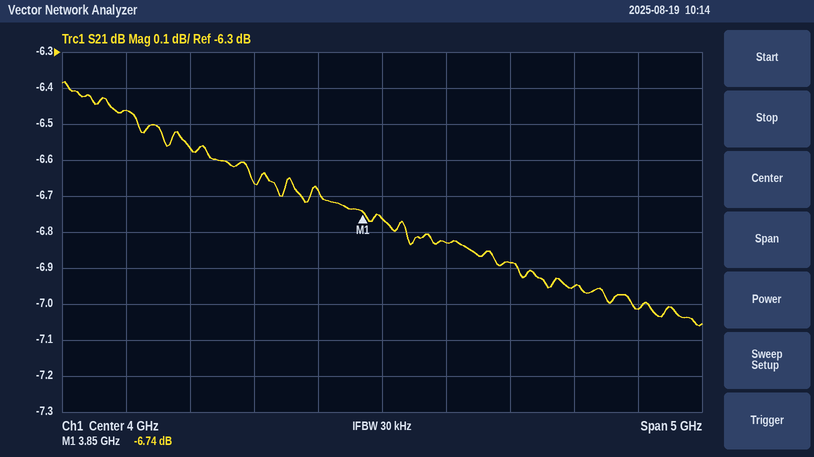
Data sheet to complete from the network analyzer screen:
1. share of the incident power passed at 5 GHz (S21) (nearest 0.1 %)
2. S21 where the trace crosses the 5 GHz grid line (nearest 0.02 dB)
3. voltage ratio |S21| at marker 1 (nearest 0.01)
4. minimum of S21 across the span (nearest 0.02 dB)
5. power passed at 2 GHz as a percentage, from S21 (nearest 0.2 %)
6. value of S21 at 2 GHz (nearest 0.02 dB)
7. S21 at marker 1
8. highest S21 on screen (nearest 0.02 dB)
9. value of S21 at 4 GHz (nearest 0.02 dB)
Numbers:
20.5 %
-6.88 dB
0.46
-7.06 dB
22.6 %
-6.46 dB
-6.74 dB
-6.38 dB
-6.76 dB
